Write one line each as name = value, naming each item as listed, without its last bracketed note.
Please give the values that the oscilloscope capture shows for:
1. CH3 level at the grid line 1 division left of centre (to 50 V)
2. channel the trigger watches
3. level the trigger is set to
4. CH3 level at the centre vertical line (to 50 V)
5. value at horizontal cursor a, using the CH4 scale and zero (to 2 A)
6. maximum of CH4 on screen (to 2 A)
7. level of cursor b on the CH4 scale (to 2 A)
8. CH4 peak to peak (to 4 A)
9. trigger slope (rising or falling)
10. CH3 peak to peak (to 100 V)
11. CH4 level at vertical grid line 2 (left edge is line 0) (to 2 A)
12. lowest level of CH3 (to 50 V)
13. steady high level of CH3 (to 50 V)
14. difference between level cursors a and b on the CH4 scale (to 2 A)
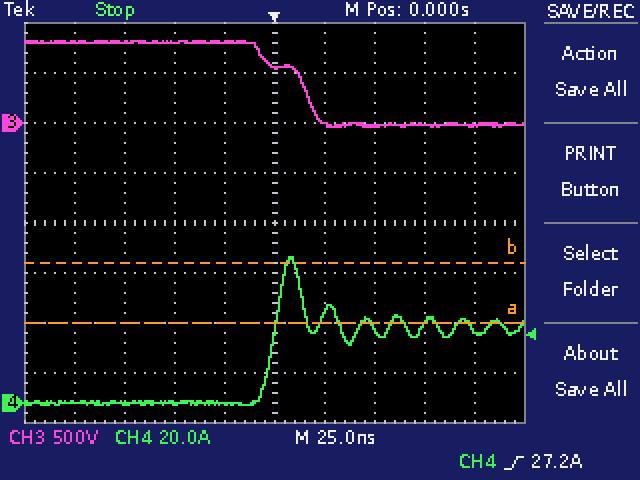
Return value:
CH3 level at the grid line 1 division left of centre = 800 V
channel the trigger watches = CH4
level the trigger is set to = 27.2 A
CH3 level at the centre vertical line = 550 V
value at horizontal cursor a, using the CH4 scale and zero = 32 A
maximum of CH4 on screen = 58 A
level of cursor b on the CH4 scale = 56 A
CH4 peak to peak = 60 A
trigger slope = rising
CH3 peak to peak = 900 V
CH4 level at vertical grid line 2 (left edge is line 0) = 0 A
lowest level of CH3 = -50 V
steady high level of CH3 = 800 V
difference between level cursors a and b on the CH4 scale = 24 A
